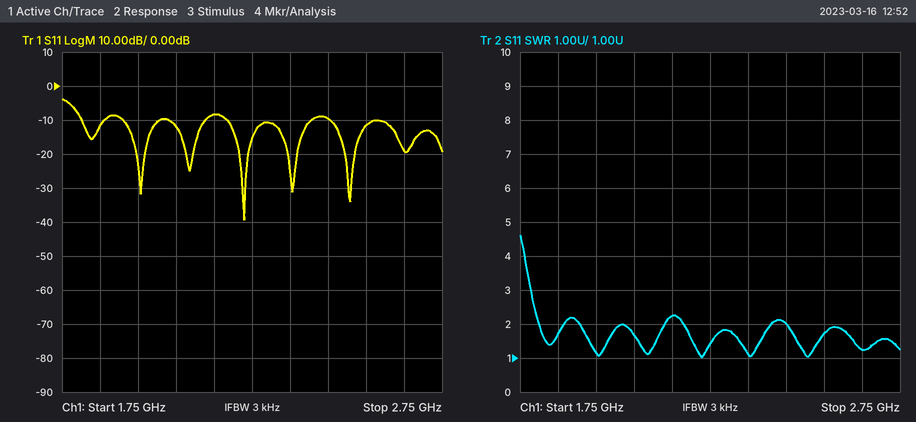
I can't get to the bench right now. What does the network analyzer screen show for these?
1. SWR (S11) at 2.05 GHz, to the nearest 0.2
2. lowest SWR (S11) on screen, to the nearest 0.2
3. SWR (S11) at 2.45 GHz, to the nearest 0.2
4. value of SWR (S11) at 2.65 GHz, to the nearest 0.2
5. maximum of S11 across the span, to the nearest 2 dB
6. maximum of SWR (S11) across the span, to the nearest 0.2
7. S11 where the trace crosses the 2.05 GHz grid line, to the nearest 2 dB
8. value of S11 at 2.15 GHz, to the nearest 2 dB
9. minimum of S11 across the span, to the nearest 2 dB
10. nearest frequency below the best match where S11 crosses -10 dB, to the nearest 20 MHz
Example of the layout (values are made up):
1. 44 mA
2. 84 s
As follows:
1. 1.6
2. 1.0
3. 2.0
4. 1.2
5. -4 dB
6. 4.6
7. -12 dB
8. -8 dB
9. -40 dB
10. 2.18 GHz
